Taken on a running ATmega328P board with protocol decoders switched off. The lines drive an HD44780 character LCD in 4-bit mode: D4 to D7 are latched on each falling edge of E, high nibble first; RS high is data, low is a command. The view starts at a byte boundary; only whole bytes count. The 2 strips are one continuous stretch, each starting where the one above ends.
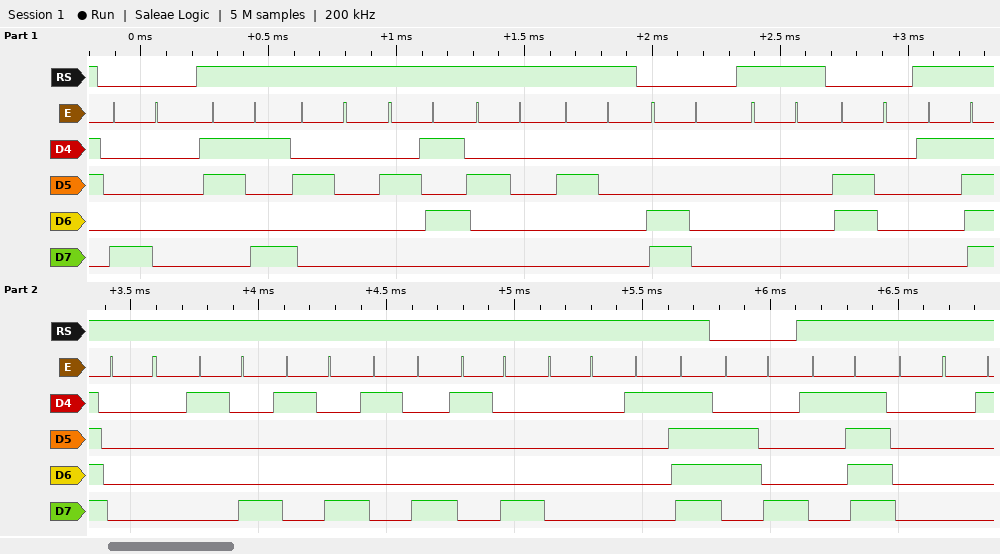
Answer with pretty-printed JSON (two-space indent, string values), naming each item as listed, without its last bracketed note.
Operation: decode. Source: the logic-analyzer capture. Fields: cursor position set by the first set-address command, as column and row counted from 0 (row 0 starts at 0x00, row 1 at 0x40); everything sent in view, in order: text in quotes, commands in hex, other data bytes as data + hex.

{
  "cursor position set by the first set-address command, as column and row counted from 0": "column 0, row 0",
  "everything sent in view, in order: text in quotes, commands in hex, other data bytes as data + hex": "0x80 \"9 %  \" 0xC0 data 00 0x60 data 1F 00 18 18 18 18 00 1F 0x68 data 1F 00"
}
